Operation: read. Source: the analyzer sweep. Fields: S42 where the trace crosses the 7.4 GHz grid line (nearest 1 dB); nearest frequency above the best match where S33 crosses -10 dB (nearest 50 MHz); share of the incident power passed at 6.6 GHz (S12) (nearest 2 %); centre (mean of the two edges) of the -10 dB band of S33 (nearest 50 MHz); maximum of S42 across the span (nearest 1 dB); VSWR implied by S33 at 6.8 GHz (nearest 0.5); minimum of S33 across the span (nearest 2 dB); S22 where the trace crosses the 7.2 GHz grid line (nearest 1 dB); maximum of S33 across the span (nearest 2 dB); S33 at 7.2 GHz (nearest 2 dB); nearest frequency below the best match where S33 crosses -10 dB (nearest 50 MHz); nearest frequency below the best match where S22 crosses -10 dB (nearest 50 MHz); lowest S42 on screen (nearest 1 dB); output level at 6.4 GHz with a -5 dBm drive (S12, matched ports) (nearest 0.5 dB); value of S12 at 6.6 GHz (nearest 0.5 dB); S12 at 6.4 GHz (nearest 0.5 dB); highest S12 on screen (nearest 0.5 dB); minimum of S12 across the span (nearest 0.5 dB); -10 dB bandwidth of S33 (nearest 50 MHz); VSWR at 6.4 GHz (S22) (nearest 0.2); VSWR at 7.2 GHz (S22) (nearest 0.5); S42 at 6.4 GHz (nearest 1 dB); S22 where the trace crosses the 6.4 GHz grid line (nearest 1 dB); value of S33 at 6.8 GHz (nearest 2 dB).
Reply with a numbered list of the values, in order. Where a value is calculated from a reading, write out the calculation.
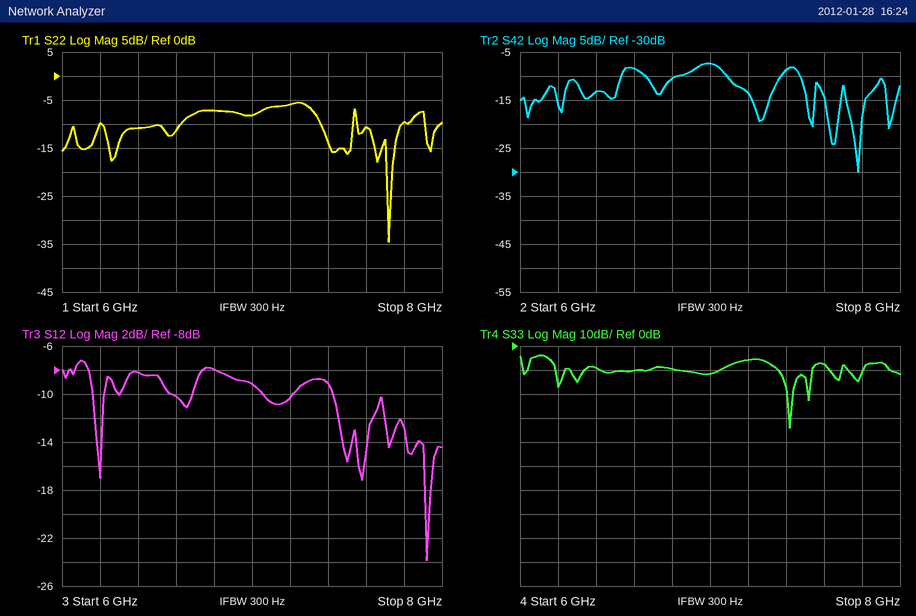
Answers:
1. -9 dB
2. 7.55 GHz
3. 10^(-10/10) ≈ 10 %
4. 7.45 GHz
5. -7 dB
6. |Γ| = 10^(-10/20) = 0.3162; VSWR = (1 + 0.3162)/(1 − 0.3162) ≈ 1.92, so 2.0 to the nearest 0.5
7. -34 dB
8. -6 dB
9. -4 dB
10. -6 dB
11. 7.35 GHz
12. 7.55 GHz
13. -30 dB
14. -5 dBm + (-8.0 dB) = -13.0 dBm
15. -10.0 dB
16. -8.0 dB
17. -7.0 dB
18. -24.0 dB
19. 7.55 GHz − 7.35 GHz = 200 MHz
20. |Γ| = 10^(-11/20) = 0.2818; VSWR = (1 + 0.2818)/(1 − 0.2818) ≈ 1.8
21. |Γ| = 10^(-6/20) = 0.5012; VSWR = (1 + 0.5012)/(1 − 0.5012) ≈ 3.0
22. -13 dB
23. -11 dB
24. -10 dB
